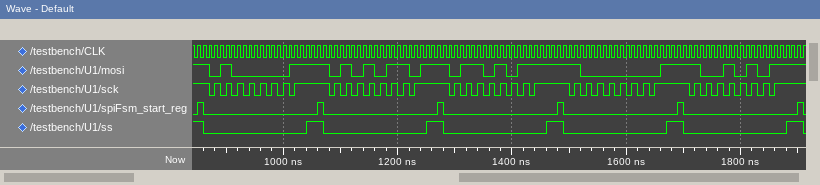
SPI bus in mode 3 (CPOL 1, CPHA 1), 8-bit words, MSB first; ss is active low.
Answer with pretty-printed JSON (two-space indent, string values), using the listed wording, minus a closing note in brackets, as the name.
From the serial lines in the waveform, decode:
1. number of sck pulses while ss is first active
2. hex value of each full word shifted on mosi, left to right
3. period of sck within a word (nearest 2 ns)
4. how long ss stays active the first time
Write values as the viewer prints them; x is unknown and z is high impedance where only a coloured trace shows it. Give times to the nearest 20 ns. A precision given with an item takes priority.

{
  "number of sck pulses while ss is first active": "8",
  "hex value of each full word shifted on mosi, left to right": "41, 56, 6B, 80, 95",
  "period of sck within a word": "20 ns",
  "how long ss stays active the first time": "180 ns"
}
